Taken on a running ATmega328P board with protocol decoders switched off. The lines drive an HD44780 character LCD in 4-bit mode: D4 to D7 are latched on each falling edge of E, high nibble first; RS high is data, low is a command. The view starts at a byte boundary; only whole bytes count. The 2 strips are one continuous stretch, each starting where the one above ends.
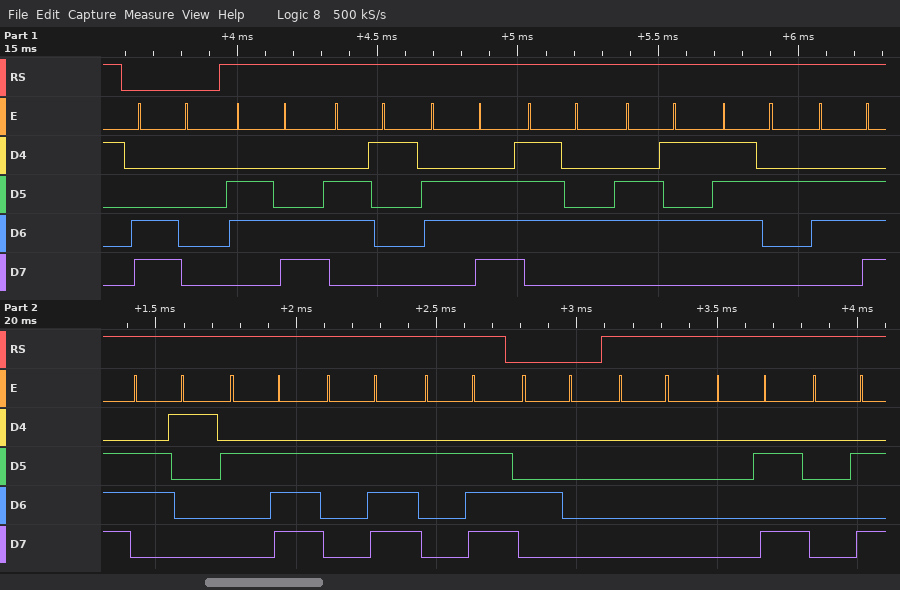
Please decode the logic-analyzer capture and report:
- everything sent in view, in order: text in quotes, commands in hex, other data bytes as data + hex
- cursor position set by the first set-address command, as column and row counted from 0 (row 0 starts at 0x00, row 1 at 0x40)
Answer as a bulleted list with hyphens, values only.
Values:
- 0xC0 "lanterna..." 0x40 data 00 0A 0A
- column 0, row 1
